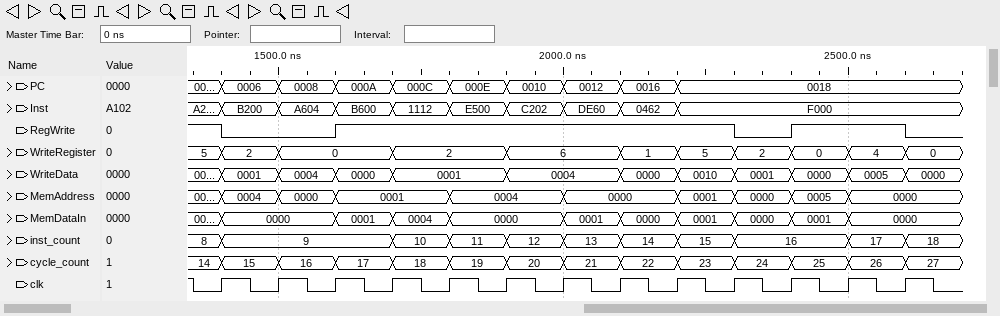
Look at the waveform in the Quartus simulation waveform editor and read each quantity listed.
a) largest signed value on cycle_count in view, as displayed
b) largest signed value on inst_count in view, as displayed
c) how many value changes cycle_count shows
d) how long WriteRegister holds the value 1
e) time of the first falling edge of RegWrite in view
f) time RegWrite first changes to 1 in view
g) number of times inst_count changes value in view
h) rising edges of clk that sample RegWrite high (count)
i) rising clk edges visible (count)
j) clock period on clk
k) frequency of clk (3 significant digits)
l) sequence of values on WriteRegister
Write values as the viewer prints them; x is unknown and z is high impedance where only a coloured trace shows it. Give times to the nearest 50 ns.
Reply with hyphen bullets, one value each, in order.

- 27
- 18
- 13
- 100 ns
- 1400 ns
- 1600 ns
- 10
- 10
- 13
- 100 ns
- 10.0 MHz
- 5, 2, 0, 2, 6, 1, 5, 2, 0, 4, 0
